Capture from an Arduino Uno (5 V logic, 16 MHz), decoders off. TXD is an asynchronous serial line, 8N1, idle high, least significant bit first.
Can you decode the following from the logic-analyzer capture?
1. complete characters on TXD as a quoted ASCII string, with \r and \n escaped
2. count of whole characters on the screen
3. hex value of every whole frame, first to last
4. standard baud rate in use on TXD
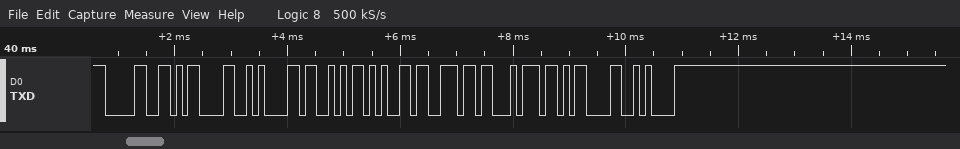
"0\r\nSent\r\n"
9
0x30 0x0D 0x0A 0x53 0x65 0x6E 0x74 0x0D 0x0A
9600 baud
